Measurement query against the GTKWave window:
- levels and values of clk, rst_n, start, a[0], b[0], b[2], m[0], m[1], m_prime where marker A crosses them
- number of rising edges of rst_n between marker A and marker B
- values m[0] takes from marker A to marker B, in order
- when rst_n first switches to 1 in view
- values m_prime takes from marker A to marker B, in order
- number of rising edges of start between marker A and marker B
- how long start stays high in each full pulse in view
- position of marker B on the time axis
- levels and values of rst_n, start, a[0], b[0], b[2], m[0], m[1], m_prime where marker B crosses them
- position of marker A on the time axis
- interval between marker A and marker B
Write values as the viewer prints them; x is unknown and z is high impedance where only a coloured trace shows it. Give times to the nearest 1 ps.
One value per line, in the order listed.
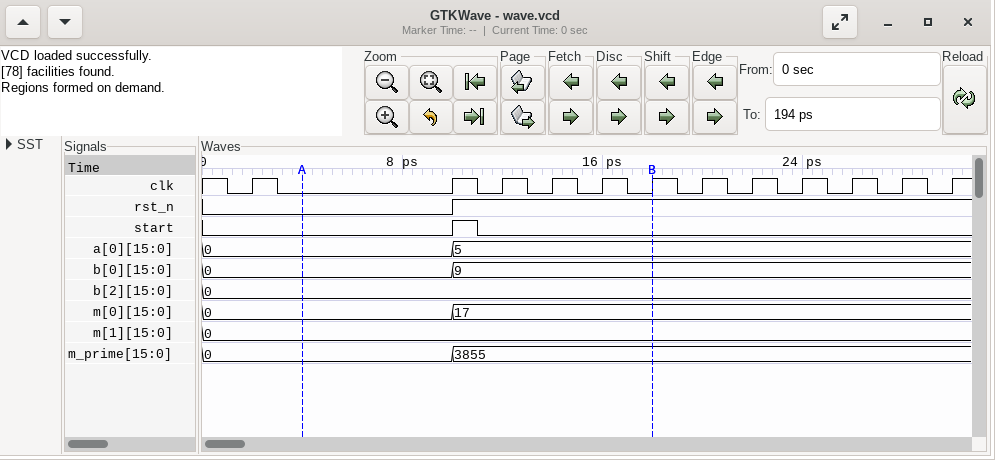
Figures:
clk=0, rst_n=0, start=0, a[0]=0, b[0]=0, b[2]=0, m[0]=0, m[1]=0, m_prime=0
1
0, 17
10 ps
0, 3855
1
1 ps
18 ps
rst_n=1, start=0, a[0]=5, b[0]=9, b[2]=0, m[0]=17, m[1]=0, m_prime=3855
4 ps
14 ps
